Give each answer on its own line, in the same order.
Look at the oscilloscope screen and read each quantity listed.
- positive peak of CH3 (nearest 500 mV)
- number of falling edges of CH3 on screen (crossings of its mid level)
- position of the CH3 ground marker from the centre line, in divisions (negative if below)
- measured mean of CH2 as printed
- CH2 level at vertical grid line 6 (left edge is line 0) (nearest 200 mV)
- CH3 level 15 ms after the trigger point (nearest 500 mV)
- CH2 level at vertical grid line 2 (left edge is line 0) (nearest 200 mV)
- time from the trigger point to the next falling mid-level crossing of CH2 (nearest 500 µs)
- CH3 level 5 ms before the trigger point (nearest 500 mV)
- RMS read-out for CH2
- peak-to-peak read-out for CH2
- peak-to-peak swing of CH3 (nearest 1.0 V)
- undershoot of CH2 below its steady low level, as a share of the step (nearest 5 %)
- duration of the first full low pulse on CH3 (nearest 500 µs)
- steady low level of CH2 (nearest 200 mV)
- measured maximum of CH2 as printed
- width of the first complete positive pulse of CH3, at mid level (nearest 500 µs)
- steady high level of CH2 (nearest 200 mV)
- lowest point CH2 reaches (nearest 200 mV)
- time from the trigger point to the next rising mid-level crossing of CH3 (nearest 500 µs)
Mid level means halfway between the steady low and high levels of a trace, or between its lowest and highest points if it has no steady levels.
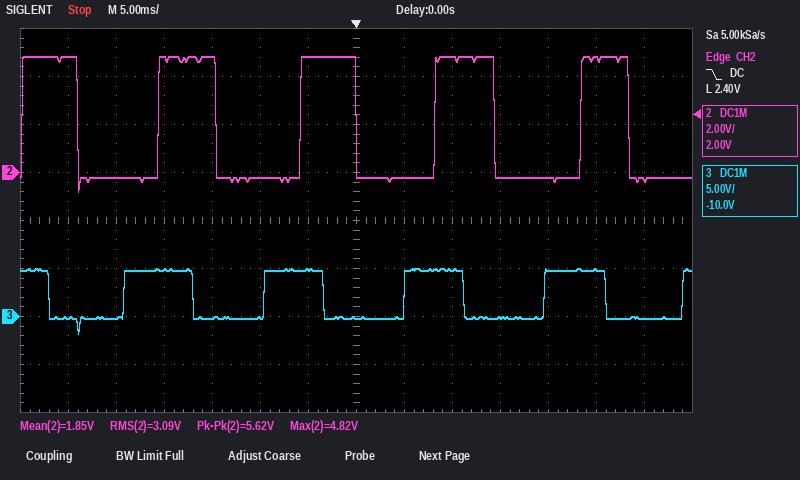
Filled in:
5.0 V
5
-2.0 div
1.85 V
4.8 V
0.0 V
-200 mV
14.5 ms
5.0 V
3.09 V
5.62 V
7.0 V
10 %
8.0 ms
-200 mV
4.82 V
7.0 ms
4.8 V
-800 mV
5.0 ms
